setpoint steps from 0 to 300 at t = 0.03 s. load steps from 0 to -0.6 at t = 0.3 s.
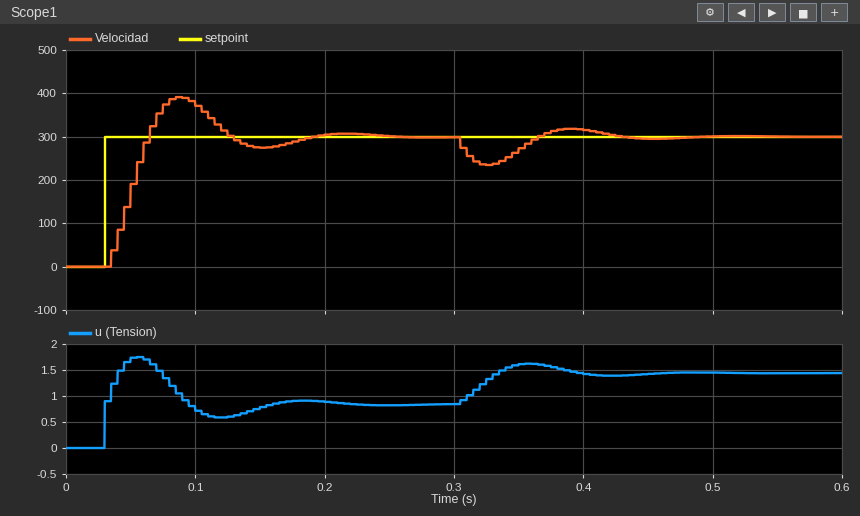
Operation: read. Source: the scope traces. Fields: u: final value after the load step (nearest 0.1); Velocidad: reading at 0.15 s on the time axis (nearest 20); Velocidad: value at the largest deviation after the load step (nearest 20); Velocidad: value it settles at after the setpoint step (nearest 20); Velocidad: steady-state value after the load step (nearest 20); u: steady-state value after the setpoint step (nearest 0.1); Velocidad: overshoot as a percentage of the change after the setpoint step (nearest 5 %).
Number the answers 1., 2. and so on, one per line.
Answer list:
1. 1.4
2. 280
3. 240
4. 300
5. 300
6. 0.8
7. 30 %
